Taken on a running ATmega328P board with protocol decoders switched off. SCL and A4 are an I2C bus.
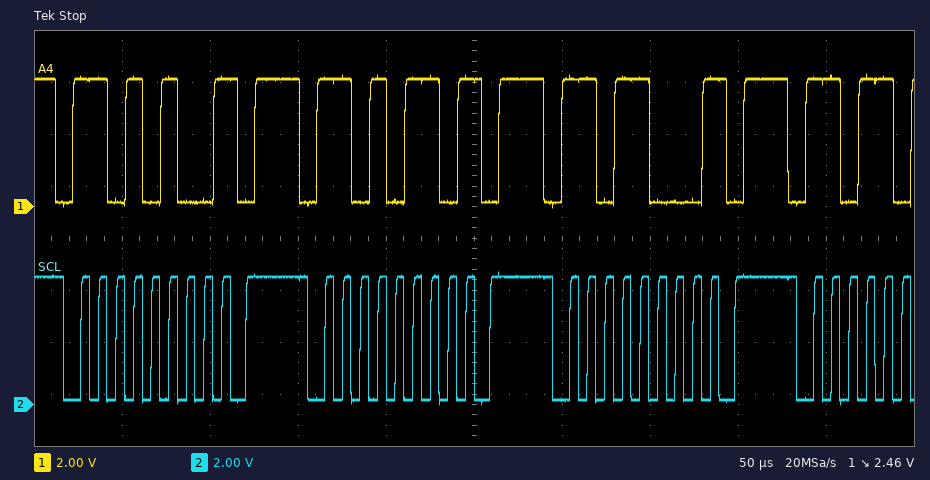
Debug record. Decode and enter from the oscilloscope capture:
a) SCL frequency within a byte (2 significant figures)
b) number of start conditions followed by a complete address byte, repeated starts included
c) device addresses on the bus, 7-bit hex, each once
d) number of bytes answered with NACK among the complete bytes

100 kHz
3
0x6A 0x6B 0x6C
3
